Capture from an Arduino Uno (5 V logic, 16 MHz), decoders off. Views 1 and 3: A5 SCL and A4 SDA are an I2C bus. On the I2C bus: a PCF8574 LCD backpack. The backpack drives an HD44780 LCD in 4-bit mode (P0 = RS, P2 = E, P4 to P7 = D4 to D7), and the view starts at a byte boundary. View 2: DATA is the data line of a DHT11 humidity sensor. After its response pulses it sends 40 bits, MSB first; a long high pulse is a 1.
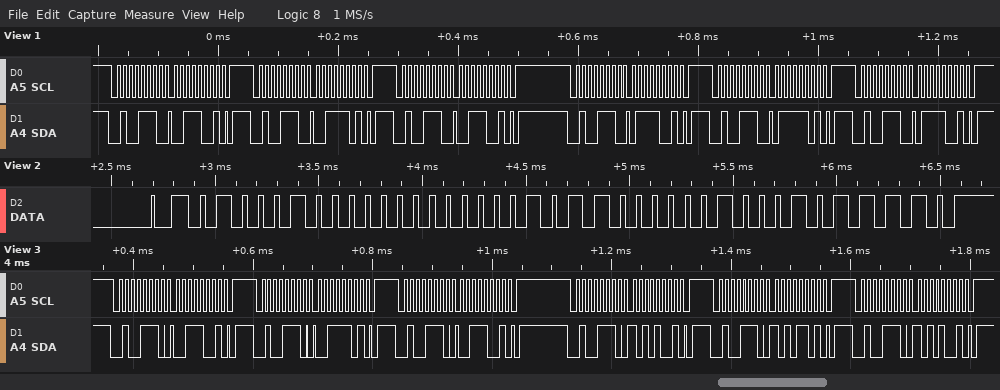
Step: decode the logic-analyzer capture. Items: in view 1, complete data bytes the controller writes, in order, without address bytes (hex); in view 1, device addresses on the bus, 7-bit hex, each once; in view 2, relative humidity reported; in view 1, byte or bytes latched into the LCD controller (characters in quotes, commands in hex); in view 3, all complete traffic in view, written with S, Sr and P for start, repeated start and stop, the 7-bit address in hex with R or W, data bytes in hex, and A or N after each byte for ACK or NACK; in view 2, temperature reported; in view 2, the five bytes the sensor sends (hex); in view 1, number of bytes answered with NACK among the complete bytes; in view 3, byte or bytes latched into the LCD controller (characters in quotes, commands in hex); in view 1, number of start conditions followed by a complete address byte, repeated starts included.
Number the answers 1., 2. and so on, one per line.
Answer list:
1. 39 3D 39 79 7D 79
2. 0x27
3. 68 %
4. '7'
5. S 27W A 39 A P S 27W A 3D A P S 27W A 39 A P S 27W A A9 A P S 27W A AD A P S 27W A A9 A P
6. 22.4 °C
7. 44 00 16 04 5E
8. 0
9. ':'
10. 6
